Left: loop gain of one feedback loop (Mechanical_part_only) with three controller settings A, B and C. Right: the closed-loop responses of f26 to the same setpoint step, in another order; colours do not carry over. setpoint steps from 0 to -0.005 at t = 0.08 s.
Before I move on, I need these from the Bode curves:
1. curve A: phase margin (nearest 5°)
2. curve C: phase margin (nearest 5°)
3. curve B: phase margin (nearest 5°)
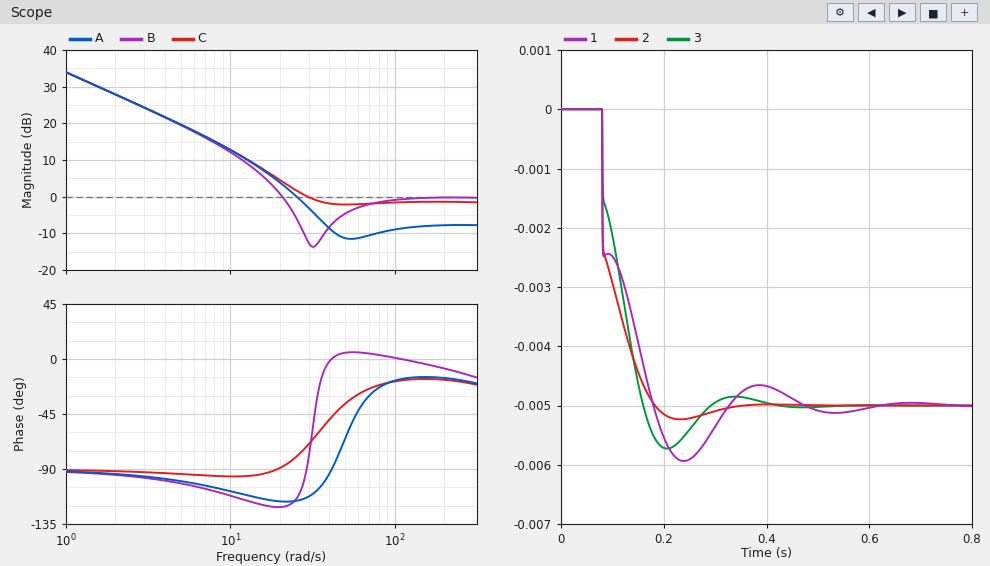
65°
110°
60°
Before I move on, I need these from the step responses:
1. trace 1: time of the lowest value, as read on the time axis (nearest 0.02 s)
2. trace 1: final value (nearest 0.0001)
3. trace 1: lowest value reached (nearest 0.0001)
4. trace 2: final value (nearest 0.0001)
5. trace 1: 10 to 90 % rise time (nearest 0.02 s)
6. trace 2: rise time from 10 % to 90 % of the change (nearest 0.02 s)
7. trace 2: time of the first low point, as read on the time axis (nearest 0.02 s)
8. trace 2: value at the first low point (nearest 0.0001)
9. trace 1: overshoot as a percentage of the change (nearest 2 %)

0.24 s
-0.0050
-0.0059
-0.0050
0.08 s
0.08 s
0.24 s
-0.0052
18 %
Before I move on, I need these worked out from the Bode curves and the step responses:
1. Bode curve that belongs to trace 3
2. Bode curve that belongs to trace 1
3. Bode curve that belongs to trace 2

A
B
C
